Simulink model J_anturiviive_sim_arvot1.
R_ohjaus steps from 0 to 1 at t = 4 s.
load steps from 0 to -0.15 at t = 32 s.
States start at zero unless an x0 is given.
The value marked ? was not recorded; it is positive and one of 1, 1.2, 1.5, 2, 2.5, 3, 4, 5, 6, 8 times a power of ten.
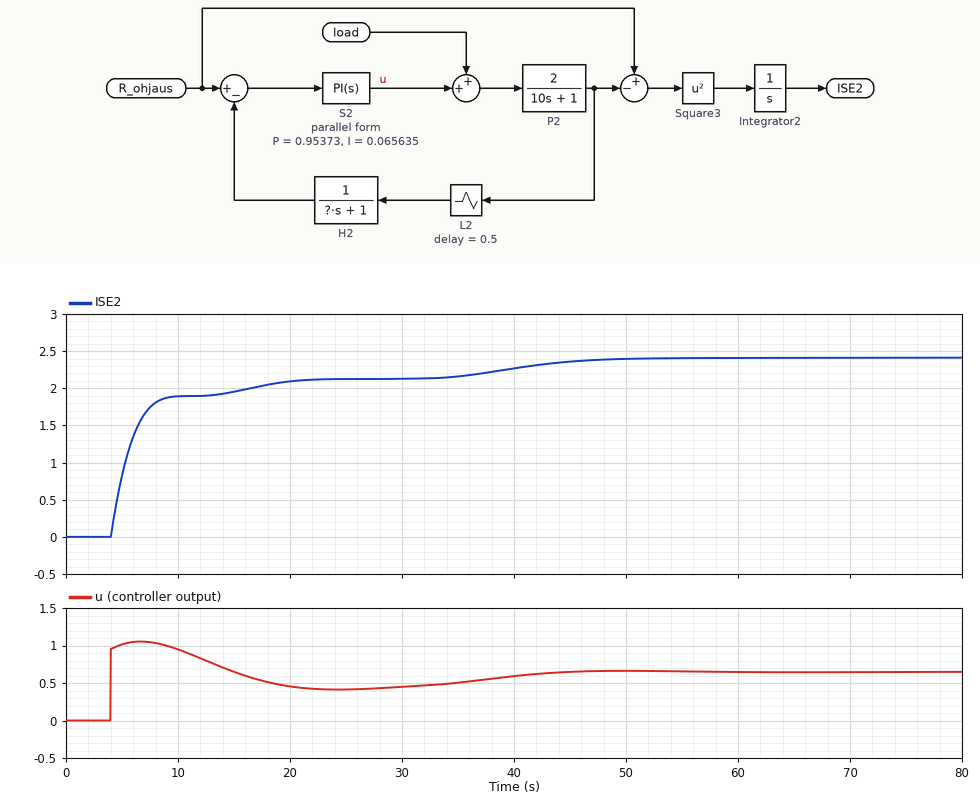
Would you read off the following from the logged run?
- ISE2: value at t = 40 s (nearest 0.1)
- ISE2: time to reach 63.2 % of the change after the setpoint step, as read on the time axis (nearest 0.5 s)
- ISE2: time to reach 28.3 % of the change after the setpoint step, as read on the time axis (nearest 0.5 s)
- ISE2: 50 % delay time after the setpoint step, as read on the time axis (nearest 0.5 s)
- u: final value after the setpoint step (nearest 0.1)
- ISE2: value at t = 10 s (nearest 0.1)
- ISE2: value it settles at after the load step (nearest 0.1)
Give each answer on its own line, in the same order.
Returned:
2.3
6.0 s
4.5 s
5.5 s
0.5
1.9
2.4
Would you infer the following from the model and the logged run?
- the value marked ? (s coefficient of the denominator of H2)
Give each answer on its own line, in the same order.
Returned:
5
